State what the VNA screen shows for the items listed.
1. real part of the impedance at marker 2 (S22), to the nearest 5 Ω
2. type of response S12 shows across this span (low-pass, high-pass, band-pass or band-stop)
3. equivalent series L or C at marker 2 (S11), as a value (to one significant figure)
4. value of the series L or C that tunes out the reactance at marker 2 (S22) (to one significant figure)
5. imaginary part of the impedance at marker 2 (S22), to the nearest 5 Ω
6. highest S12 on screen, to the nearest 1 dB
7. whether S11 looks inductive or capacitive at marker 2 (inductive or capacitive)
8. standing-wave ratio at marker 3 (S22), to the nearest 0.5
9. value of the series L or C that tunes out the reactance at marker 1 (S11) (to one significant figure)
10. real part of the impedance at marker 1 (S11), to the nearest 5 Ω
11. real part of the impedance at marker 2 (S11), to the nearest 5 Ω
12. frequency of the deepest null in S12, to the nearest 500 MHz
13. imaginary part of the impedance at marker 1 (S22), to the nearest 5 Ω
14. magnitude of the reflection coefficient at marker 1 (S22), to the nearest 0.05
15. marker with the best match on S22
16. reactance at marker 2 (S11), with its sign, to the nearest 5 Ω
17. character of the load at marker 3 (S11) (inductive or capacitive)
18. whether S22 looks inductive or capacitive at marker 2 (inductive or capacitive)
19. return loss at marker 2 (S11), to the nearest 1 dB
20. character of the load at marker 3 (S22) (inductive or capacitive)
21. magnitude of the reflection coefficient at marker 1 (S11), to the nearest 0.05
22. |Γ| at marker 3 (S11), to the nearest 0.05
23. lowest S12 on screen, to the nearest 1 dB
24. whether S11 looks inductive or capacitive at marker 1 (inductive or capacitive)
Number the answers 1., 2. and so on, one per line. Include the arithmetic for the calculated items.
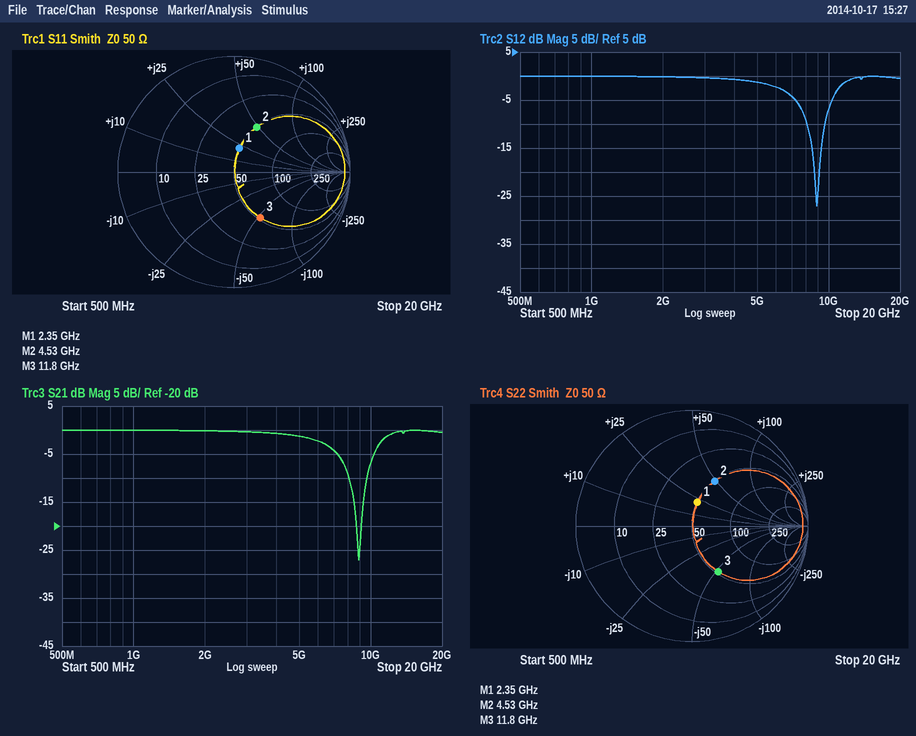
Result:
1. 50 Ω
2. band-stop
3. L = 50 Ω/(2π × 4.53 GHz) ≈ 2 nH
4. C = 1/(2π × 4.53 GHz × 50 Ω) ≈ 703 fF, so 700 fF to one significant figure
5. +50 Ω
6. 0 dB
7. inductive
8. 2.5
9. C = 1/(2π × 2.35 GHz × 20 Ω) ≈ 3 pF
10. 50 Ω
11. 50 Ω
12. 9.0 GHz
13. +20 Ω
14. 0.20
15. marker 1
16. +50 Ω
17. capacitive
18. inductive
19. 7 dB
20. capacitive
21. 0.20
22. 0.45
23. -27 dB
24. inductive
